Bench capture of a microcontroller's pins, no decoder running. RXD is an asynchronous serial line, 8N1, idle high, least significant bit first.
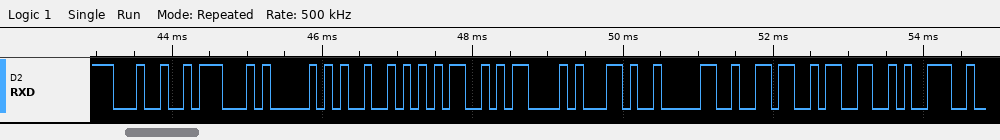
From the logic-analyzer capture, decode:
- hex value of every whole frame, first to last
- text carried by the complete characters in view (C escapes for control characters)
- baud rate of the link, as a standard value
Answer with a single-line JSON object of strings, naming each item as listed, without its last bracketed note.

{"hex value of every whole frame, first to last": "0x24 0x47 0x50 0x52 0x4D 0x43 0x2C 0x30 0x36 0x33 0x39", "text carried by the complete characters in view": "\"$GPRMC,0639\"", "baud rate of the link, as a standard value": "9600 baud"}
